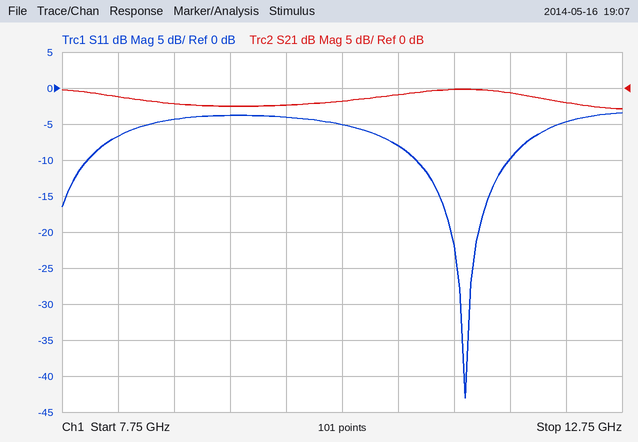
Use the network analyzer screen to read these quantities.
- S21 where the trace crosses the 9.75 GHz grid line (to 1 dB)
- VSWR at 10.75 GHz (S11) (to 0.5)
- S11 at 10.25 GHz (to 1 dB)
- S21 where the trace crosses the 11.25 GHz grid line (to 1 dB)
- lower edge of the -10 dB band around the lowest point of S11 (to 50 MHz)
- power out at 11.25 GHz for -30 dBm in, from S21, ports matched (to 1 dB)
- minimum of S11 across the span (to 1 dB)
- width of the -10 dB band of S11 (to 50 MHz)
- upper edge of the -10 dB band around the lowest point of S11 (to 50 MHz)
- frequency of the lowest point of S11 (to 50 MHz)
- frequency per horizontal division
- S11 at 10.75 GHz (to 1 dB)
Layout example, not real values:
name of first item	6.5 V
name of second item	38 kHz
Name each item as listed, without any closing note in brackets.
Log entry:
S21 where the trace crosses the 9.75 GHz grid line	-2 dB
VSWR at 10.75 GHz (S11)	2.5
S11 at 10.25 GHz	-5 dB
S21 where the trace crosses the 11.25 GHz grid line	0 dB
lower edge of the -10 dB band around the lowest point of S11	10.90 GHz
power out at 11.25 GHz for -30 dBm in, from S21, ports matched	-30 dBm
minimum of S11 across the span	-43 dB
width of the -10 dB band of S11	850 MHz
upper edge of the -10 dB band around the lowest point of S11	11.75 GHz
frequency of the lowest point of S11	11.35 GHz
frequency per horizontal division	500 MHz
S11 at 10.75 GHz	-8 dB
